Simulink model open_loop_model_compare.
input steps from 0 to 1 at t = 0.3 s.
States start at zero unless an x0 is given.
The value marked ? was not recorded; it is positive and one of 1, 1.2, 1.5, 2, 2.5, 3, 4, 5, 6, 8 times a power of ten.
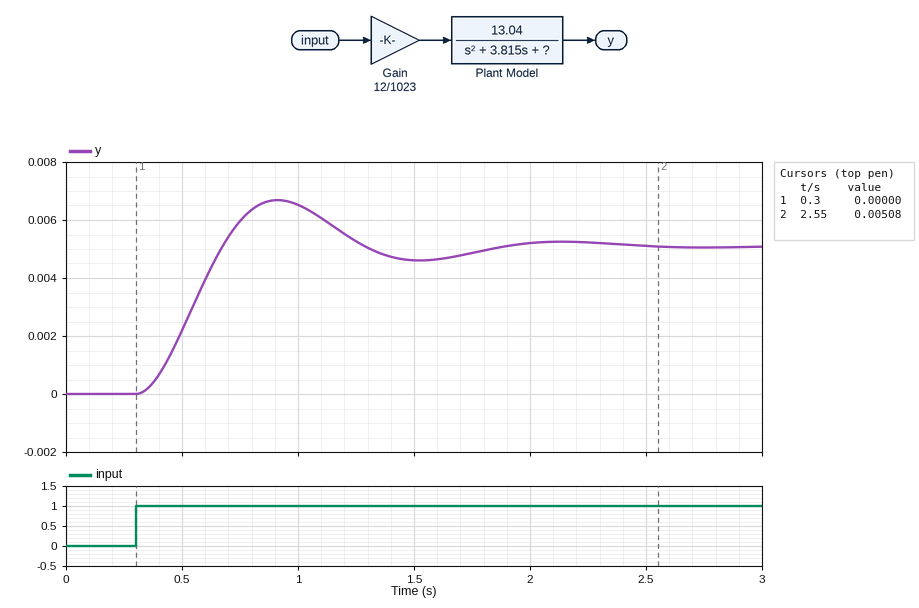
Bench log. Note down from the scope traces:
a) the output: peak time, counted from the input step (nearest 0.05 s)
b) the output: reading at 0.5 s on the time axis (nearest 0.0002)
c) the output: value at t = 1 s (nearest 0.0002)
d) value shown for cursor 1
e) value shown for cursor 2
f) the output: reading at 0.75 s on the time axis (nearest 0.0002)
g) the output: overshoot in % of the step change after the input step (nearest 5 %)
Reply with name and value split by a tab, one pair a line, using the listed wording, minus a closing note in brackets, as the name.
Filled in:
the output: peak time, counted from the input step	0.60 s
the output: reading at 0.5 s on the time axis	0.0022
the output: value at t = 1 s	0.0066
value shown for cursor 1	0.00000
value shown for cursor 2	0.00508
the output: reading at 0.75 s on the time axis	0.0060
the output: overshoot in % of the step change after the input step	30 %
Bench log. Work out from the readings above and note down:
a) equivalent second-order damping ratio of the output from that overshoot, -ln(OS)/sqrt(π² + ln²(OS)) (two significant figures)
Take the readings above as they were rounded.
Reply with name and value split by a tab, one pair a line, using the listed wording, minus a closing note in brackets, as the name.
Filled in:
equivalent second-order damping ratio of the output from that overshoot, -ln(OS)/sqrt(π² + ln²(OS))	0.36
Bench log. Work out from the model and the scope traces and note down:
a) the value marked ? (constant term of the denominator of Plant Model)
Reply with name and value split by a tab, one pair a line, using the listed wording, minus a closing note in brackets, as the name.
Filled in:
the value marked ?	30
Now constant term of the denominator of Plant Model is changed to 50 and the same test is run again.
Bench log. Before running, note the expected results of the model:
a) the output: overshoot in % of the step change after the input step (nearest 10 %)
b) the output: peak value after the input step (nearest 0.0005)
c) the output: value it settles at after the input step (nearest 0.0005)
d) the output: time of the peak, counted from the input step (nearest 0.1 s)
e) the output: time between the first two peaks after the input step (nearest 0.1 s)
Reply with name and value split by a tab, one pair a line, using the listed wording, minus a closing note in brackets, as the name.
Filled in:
the output: overshoot in % of the step change after the input step	40 %
the output: peak value after the input step	0.0045
the output: value it settles at after the input step	0.0030
the output: time of the peak, counted from the input step	0.5 s
the output: time between the first two peaks after the input step	0.9 s
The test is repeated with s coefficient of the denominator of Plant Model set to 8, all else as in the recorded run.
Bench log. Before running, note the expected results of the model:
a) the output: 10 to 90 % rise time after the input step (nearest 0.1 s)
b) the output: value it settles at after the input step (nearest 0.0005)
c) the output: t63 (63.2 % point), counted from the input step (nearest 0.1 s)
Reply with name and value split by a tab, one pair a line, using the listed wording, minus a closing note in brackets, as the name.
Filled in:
the output: 10 to 90 % rise time after the input step	0.4 s
the output: value it settles at after the input step	0.0050
the output: t63 (63.2 % point), counted from the input step	0.3 s
